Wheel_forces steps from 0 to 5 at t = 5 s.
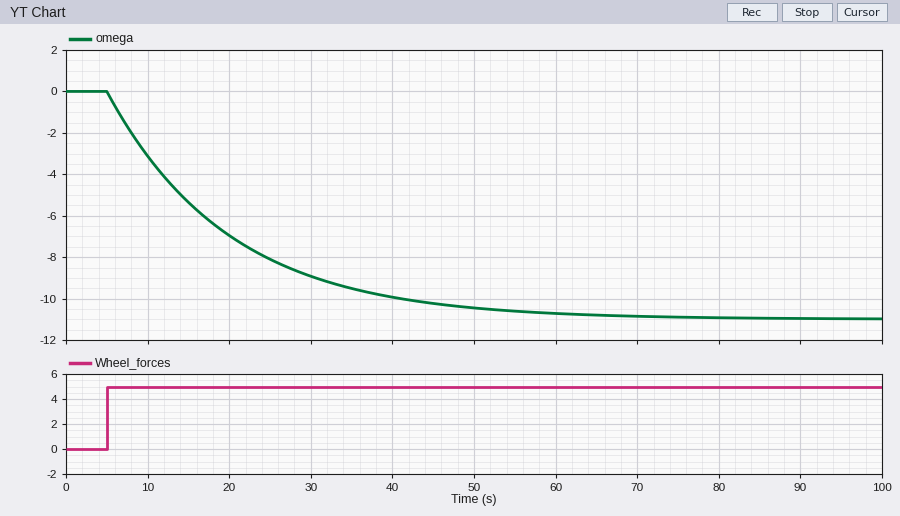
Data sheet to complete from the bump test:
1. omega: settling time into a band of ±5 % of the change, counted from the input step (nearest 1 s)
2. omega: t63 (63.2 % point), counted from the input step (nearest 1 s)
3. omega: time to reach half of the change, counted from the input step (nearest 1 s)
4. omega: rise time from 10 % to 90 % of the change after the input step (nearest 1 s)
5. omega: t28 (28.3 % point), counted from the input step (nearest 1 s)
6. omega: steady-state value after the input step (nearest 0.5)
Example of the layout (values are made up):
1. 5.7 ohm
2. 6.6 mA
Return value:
1. 45 s
2. 15 s
3. 10 s
4. 33 s
5. 5 s
6. -11.0
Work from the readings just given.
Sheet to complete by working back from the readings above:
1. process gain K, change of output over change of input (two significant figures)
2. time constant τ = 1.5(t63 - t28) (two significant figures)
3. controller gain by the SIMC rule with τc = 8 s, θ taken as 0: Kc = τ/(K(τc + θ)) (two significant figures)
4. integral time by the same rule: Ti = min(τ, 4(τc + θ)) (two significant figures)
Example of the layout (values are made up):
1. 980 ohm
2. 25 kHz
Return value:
1. -2.2
2. 15 s
3. -0.85
4. 15 s
